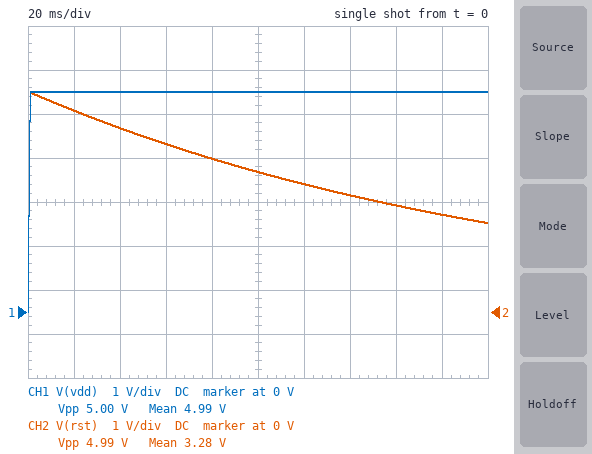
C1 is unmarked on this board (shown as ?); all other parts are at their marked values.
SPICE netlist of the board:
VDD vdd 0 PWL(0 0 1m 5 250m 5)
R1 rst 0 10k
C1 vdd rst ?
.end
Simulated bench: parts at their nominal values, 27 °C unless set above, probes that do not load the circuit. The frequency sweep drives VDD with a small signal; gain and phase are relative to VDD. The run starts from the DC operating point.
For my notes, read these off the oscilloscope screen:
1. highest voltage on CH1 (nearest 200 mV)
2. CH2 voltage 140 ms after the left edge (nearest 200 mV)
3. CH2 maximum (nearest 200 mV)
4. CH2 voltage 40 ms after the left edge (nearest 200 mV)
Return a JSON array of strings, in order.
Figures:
["5.0 V", "2.6 V", "5.0 V", "4.2 V"]
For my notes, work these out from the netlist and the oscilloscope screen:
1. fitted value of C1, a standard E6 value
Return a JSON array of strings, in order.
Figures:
["22 µF"]
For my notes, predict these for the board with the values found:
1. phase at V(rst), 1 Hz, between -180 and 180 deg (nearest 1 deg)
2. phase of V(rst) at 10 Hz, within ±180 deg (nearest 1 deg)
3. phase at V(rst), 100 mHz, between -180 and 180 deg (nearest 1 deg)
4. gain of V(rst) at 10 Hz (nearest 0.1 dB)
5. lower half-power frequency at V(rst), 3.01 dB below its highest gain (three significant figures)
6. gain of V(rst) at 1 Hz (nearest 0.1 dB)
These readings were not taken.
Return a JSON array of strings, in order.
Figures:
["36 deg", "4 deg", "82 deg", "0 dB", "723 mHz", "-1.8 dB"]
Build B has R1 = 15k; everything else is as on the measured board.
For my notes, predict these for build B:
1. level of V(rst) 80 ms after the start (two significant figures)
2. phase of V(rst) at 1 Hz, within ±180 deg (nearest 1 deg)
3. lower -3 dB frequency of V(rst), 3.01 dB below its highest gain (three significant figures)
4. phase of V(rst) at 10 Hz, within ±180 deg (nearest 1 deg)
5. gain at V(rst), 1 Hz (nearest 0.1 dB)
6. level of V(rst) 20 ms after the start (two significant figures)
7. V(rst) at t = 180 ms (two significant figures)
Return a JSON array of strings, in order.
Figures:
["3.9 V", "26 deg", "482 mHz", "3 deg", "-0.9 dB", "4.7 V", "2.9 V"]
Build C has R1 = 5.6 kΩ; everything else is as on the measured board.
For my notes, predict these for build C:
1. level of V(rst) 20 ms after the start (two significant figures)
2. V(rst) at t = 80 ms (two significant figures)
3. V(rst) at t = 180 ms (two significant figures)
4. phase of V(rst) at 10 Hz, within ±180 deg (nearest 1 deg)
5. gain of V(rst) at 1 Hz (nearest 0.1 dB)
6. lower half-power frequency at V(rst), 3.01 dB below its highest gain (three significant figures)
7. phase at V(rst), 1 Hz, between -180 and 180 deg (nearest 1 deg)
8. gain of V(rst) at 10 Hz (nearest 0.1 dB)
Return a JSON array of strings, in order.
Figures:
["4.3 V", "2.6 V", "1.2 V", "7 deg", "-4.3 dB", "1.29 Hz", "52 deg", "-0.1 dB"]
